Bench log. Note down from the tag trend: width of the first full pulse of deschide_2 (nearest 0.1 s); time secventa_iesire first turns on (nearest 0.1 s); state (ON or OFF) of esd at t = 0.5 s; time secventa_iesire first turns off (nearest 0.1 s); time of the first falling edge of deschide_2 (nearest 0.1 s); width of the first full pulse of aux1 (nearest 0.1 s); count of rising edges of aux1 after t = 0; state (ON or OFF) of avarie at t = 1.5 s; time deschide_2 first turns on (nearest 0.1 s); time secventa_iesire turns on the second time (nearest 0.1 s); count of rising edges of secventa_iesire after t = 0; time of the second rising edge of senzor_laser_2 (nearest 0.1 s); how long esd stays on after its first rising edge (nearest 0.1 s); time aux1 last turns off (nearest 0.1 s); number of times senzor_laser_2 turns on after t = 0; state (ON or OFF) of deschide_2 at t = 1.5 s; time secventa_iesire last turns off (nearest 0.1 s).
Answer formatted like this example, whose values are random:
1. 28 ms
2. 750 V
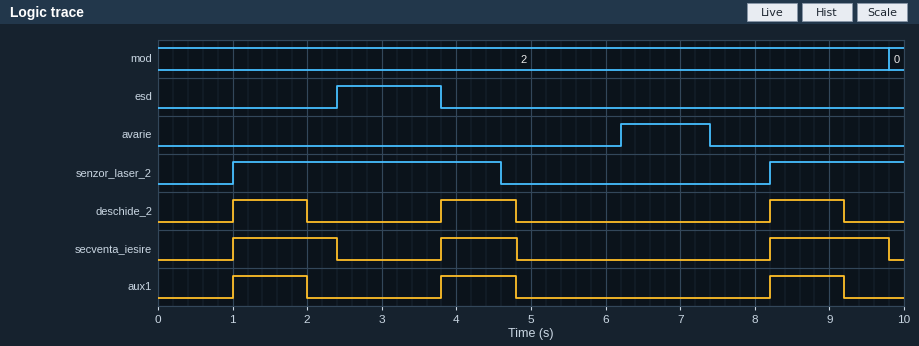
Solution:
1. 1.0 s
2. 1.0 s
3. OFF
4. 2.4 s
5. 2.0 s
6. 1.0 s
7. 3
8. OFF
9. 1.0 s
10. 3.8 s
11. 3
12. 8.2 s
13. 1.4 s
14. 9.2 s
15. 2
16. ON
17. 9.8 s
